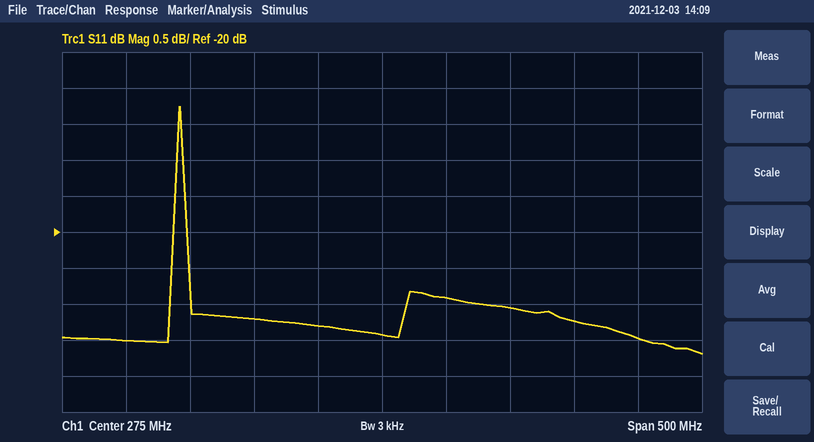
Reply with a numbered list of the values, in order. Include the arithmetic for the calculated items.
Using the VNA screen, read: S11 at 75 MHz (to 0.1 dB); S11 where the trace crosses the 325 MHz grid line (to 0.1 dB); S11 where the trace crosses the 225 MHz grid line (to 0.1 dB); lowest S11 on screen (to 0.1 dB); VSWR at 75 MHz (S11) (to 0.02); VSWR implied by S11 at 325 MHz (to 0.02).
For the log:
1. -21.5 dB
2. -20.9 dB
3. -21.3 dB
4. -21.7 dB
5. |Γ| = 10^(-21.5/20) = 0.0841; VSWR = (1 + 0.0841)/(1 − 0.0841) ≈ 1.18
6. |Γ| = 10^(-20.9/20) = 0.0902; VSWR = (1 + 0.0902)/(1 − 0.0902) ≈ 1.20
